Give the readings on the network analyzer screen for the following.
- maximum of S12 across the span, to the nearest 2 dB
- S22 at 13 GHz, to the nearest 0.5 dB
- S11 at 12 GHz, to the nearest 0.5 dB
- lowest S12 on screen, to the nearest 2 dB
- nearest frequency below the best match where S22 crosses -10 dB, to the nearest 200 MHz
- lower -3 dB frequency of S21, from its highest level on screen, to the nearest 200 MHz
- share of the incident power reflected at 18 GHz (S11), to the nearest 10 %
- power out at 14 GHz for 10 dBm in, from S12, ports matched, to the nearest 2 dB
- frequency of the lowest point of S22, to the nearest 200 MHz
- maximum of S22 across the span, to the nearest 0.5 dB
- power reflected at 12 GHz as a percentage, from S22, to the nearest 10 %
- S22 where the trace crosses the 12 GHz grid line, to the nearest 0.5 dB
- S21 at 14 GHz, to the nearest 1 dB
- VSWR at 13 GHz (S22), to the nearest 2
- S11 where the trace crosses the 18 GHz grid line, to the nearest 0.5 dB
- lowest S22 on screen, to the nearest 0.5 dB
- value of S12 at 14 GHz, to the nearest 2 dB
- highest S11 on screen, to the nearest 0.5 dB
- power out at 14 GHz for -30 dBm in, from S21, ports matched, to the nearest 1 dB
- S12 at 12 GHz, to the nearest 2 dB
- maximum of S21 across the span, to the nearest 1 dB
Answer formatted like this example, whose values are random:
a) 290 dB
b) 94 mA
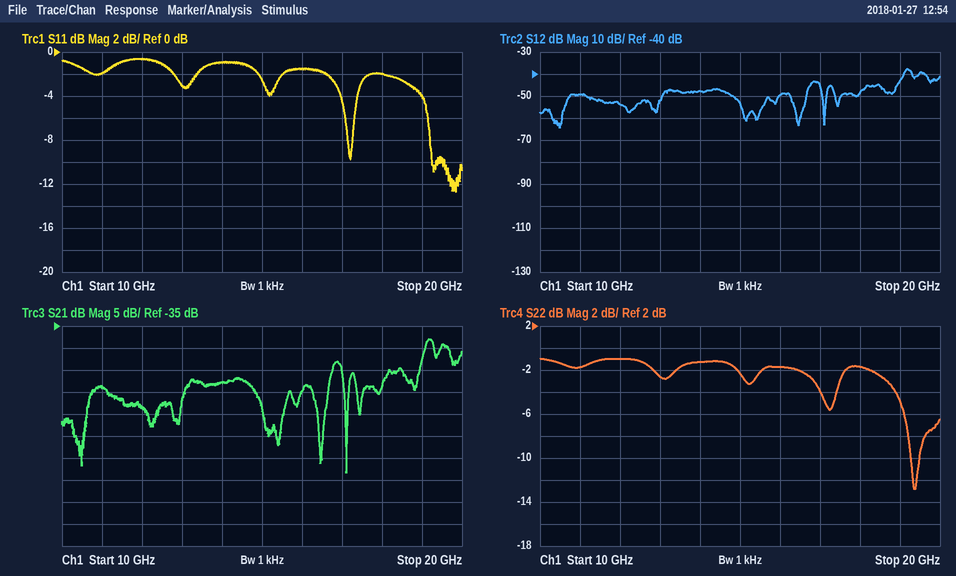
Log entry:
a) -38 dB
b) -2.5 dB
c) -0.5 dB
d) -64 dB
e) 19.2 GHz
f) 19.0 GHz
g) 60 %
h) -38 dBm
i) 19.4 GHz
j) -1.0 dB
k) 80 %
l) -1.0 dB
m) -48 dB
n) 6
o) -2.0 dB
p) -13.0 dB
q) -48 dB
r) -0.5 dB
s) -78 dBm
t) -54 dB
u) -38 dB
